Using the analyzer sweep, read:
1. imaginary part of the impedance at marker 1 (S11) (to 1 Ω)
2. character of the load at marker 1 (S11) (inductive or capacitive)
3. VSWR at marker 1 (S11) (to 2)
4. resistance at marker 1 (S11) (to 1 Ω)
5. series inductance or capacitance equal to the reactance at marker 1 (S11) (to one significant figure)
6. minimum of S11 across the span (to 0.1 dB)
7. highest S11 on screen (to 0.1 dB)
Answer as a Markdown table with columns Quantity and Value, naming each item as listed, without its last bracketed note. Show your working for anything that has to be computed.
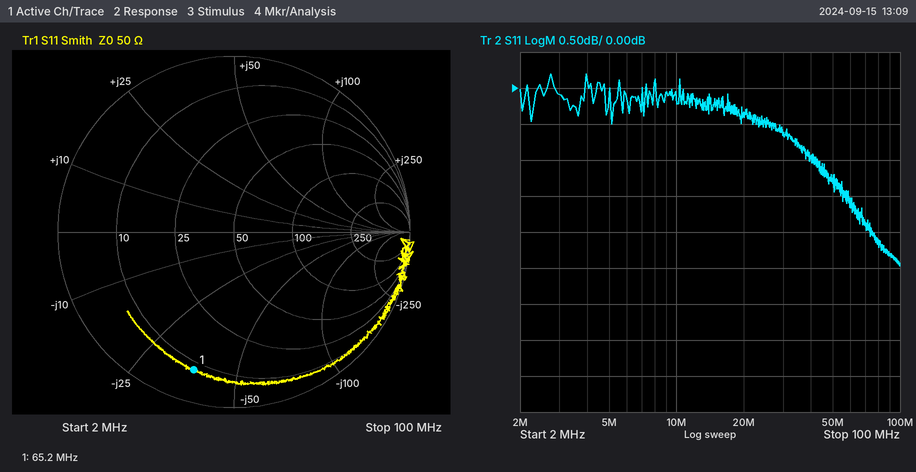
| Quantity | Value |
|---|---|
| imaginary part of the impedance at marker 1 (S11) | -37 Ω |
| character of the load at marker 1 (S11) | capacitive |
| VSWR at marker 1 (S11) | 10 |
| resistance at marker 1 (S11) | 8 Ω |
| series inductance or capacitance equal to the reactance at marker 1 (S11) | C = 1/(2π × 65.2 MHz × 37 Ω) ≈ 66.0 pF, so 70 pF to one significant figure |
| minimum of S11 across the span | -2.5 dB |
| highest S11 on screen | 0.2 dB |
